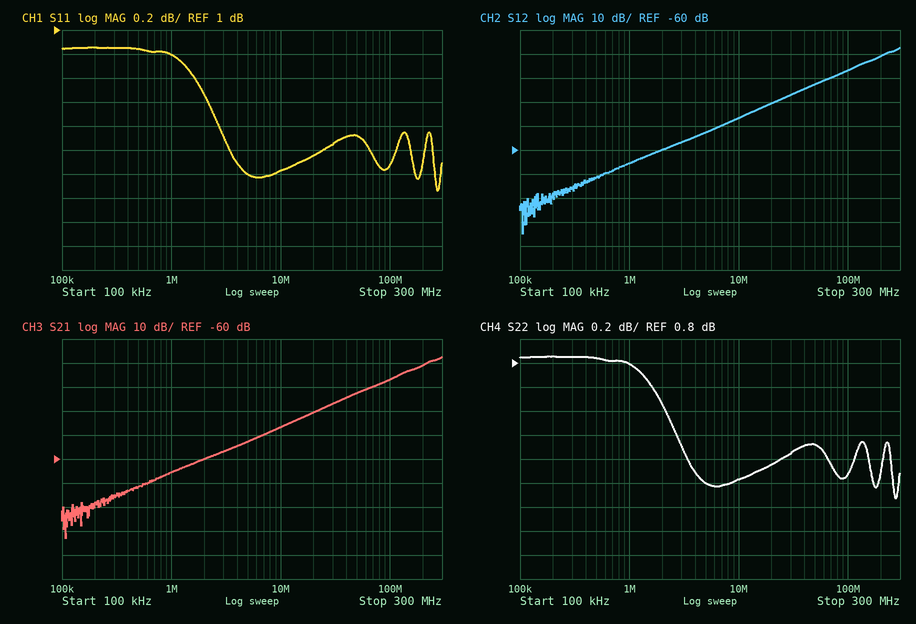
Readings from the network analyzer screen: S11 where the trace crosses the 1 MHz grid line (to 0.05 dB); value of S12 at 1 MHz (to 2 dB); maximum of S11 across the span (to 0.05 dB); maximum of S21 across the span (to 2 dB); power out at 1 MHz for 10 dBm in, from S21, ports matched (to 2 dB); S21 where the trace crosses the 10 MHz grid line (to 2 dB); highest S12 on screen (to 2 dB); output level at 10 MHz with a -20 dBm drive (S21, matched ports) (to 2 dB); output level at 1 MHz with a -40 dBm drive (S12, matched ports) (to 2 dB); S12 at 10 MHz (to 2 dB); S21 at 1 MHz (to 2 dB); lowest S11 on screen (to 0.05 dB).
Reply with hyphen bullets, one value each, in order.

- 0.80 dB
- -66 dB
- 0.85 dB
- -18 dB
- -56 dBm
- -46 dB
- -18 dB
- -66 dBm
- -106 dBm
- -46 dB
- -66 dB
- -0.35 dB
